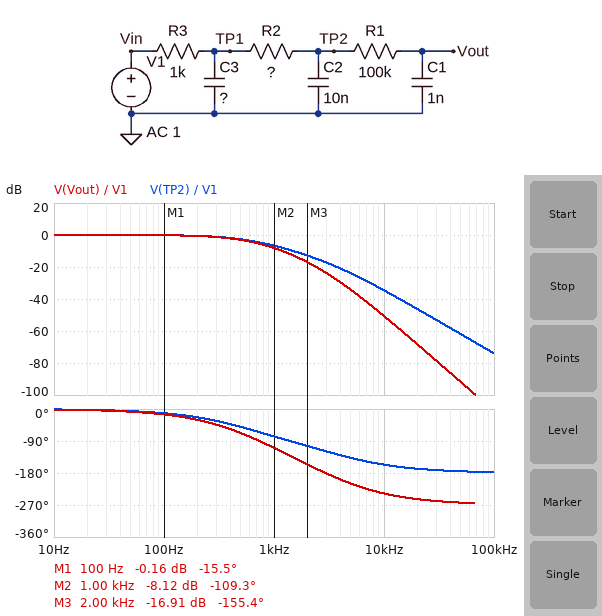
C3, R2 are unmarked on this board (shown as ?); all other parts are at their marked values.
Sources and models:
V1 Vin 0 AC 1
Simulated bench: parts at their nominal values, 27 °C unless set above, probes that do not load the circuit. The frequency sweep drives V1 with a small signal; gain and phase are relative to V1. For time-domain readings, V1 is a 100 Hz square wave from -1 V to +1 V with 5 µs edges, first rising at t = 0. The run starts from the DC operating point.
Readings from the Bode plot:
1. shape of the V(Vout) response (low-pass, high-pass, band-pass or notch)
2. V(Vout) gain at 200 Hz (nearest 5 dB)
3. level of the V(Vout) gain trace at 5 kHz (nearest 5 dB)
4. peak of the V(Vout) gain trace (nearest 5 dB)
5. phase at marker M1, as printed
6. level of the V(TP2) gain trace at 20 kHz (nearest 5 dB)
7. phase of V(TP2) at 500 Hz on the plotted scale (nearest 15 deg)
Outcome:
low-pass
0 dB
-35 dB
0 dB
-15.5 deg
-45 dB
-45 deg
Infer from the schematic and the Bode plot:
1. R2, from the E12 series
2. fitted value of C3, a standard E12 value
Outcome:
4.7 kΩ
270 nF
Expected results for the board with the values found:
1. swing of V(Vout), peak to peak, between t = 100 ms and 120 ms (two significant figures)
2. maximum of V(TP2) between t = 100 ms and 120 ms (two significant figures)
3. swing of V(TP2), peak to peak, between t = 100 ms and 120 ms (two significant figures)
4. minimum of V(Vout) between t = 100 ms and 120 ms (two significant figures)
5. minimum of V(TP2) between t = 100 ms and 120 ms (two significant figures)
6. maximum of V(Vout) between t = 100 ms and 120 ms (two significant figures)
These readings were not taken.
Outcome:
2.0 V
1.0 V
2.0 V
-1.0 V
-1.0 V
1.0 V
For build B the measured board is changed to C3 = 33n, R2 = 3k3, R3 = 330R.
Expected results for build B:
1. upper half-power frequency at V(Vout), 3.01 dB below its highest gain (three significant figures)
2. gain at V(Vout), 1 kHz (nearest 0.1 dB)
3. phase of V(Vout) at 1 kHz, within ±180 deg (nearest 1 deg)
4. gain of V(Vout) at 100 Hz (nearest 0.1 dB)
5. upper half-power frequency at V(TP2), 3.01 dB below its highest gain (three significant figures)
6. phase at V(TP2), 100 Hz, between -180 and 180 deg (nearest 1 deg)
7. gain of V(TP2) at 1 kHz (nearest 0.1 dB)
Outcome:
1.36 kHz
-1.8 dB
-50 deg
0 dB
3.81 kHz
-2 deg
-0.4 dB
